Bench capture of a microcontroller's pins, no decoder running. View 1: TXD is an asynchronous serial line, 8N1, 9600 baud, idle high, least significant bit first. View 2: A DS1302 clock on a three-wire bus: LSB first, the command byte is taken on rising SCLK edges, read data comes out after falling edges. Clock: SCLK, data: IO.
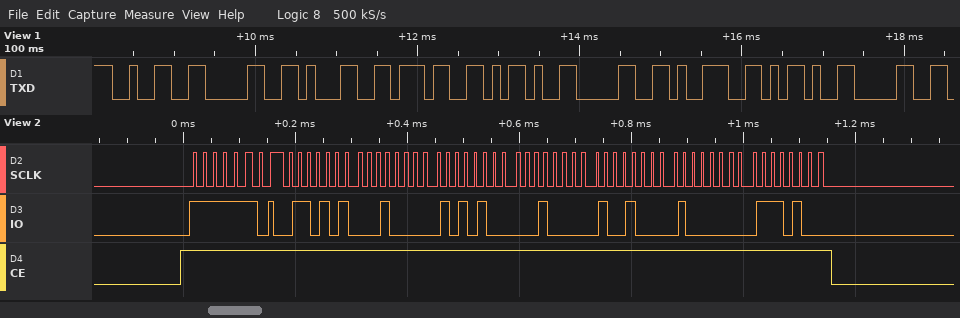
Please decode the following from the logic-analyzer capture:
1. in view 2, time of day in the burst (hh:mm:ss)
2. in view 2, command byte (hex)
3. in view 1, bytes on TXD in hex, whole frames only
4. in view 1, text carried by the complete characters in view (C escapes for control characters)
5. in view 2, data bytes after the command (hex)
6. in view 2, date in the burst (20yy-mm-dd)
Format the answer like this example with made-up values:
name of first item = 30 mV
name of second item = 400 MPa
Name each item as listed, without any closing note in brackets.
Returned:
in view 2, time of day in the burst = 15:04:56
in view 2, command byte = 0xBF
in view 1, bytes on TXD in hex, whole frames only = 0x32 0x30 0x31 0x37 0x2D 0x30 0x39 0x2D 0x30
in view 1, text carried by the complete characters in view = "2017-09-0"
in view 2, data bytes after the command = 56 04 15 04 09 01 17
in view 2, date in the burst = 2017-09-04
